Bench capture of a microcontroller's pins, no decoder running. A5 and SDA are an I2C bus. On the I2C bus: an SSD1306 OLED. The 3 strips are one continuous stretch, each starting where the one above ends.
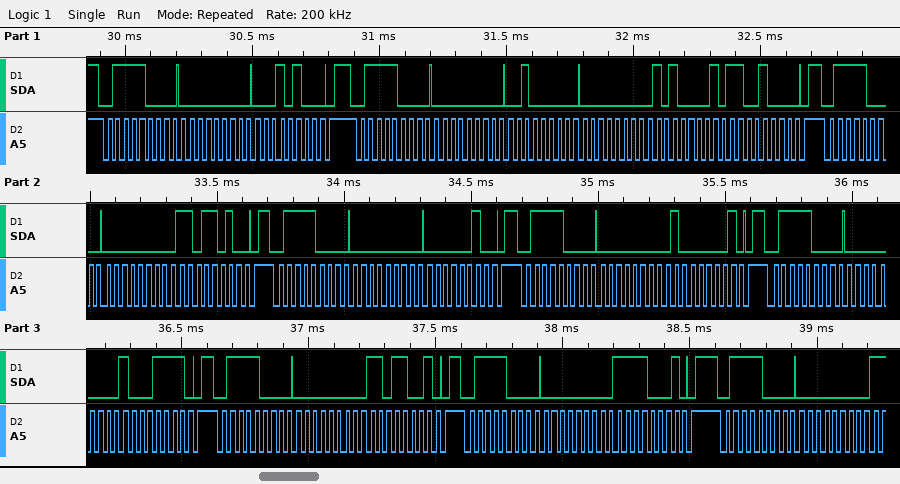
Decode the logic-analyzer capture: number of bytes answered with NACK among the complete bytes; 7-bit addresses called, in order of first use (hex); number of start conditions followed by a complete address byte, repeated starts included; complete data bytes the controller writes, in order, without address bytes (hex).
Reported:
0
0x3C
9
00 14 00 20 00 A1 C8 00 DA 00 02 00 81 00 8F 00 D9 00 F1 00
